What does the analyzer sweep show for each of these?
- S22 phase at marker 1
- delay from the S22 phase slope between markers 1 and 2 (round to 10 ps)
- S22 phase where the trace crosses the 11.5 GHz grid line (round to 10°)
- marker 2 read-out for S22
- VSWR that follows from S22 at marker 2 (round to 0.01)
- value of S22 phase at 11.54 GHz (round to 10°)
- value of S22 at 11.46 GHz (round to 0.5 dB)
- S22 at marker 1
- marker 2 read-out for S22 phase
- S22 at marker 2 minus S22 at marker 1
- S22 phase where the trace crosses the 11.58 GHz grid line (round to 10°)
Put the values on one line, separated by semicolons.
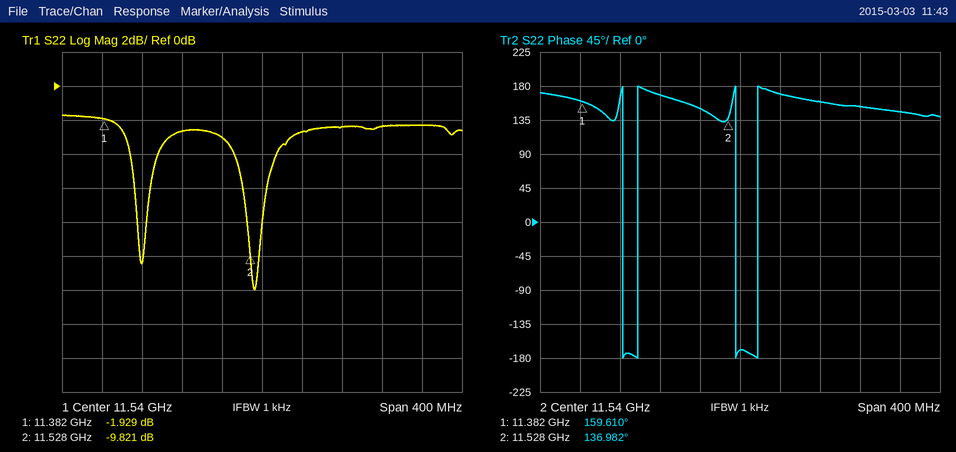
159.610°; 430 ps; 150°; -9.821 dB; 1.95; -170°; -2.5 dB; -1.929 dB; 136.982°; -7.892 dB; 170°
